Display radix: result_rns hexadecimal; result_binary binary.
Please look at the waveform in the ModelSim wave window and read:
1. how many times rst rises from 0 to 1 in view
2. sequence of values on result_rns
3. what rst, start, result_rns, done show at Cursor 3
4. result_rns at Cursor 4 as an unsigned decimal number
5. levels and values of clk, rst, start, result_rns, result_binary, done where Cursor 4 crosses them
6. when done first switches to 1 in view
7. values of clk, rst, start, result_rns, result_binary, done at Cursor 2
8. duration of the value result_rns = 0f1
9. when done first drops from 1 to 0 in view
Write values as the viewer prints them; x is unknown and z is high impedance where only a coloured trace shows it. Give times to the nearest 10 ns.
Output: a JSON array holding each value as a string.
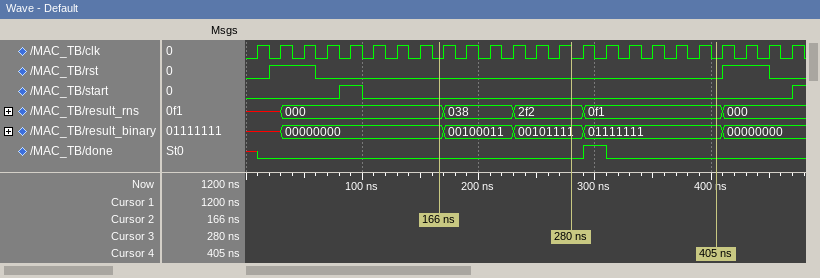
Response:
["2", "x, 000, 038, 2f2, 0f1, 000", "rst=0, start=0, result_rns=2f2, done=0", "241", "clk=0, rst=0, start=0, result_rns=0f1, result_binary=01111111, done=0", "290 ns", "clk=0, rst=0, start=0, result_rns=000, result_binary=00000000, done=0", "120 ns", "310 ns"]
